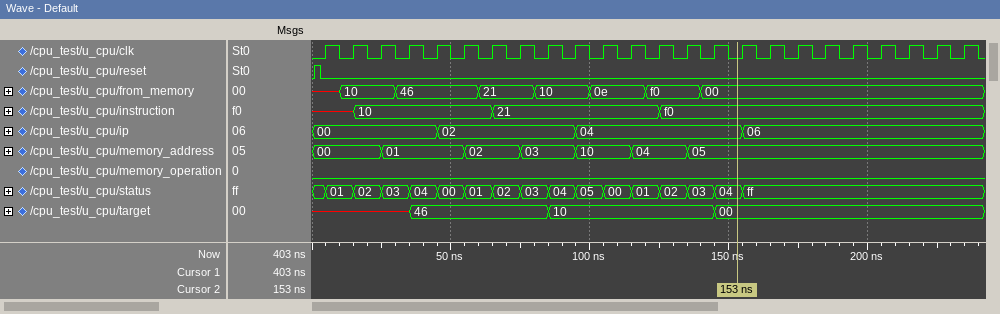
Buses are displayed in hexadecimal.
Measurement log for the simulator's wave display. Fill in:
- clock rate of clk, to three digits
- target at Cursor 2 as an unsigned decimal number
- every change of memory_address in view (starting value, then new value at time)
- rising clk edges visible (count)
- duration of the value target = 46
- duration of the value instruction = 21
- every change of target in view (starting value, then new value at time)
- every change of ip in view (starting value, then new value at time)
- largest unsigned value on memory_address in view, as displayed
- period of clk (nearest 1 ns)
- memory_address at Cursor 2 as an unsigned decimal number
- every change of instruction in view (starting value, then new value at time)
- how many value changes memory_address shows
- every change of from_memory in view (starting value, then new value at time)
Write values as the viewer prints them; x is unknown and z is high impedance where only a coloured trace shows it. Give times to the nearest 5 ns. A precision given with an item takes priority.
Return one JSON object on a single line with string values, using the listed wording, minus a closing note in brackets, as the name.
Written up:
{"clock rate of clk, to three digits": "100 MHz", "target at Cursor 2 as an unsigned decimal number": "0", "every change of memory_address in view": "00, 01 at 25 ns, 02 at 55 ns, 03 at 75 ns, 10 at 95 ns, 04 at 115 ns, 05 at 135 ns", "rising clk edges visible": "24", "duration of the value target = 46": "50 ns", "duration of the value instruction = 21": "60 ns", "every change of target in view": "x, 46 at 35 ns, 10 at 85 ns, 00 at 145 ns", "every change of ip in view": "00, 02 at 45 ns, 04 at 95 ns, 06 at 155 ns", "largest unsigned value on memory_address in view, as displayed": "10", "period of clk": "10 ns", "memory_address at Cursor 2 as an unsigned decimal number": "5", "every change of instruction in view": "x, 10 at 15 ns, 21 at 65 ns, f0 at 125 ns", "how many value changes memory_address shows": "6", "every change of from_memory in view": "x, 10 at 10 ns, 46 at 30 ns, 21 at 60 ns, 10 at 80 ns, 0e at 100 ns, f0 at 120 ns, 00 at 140 ns"}
